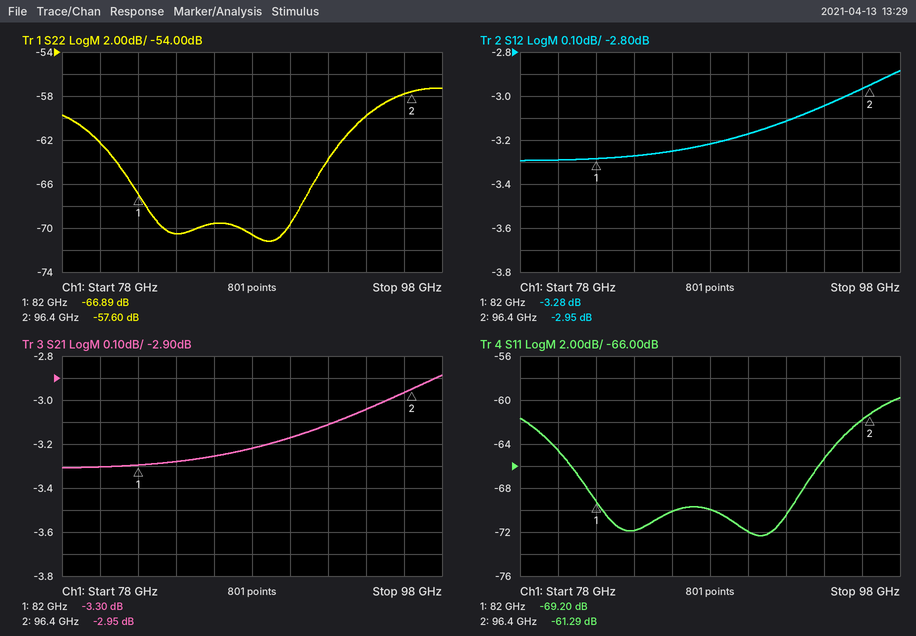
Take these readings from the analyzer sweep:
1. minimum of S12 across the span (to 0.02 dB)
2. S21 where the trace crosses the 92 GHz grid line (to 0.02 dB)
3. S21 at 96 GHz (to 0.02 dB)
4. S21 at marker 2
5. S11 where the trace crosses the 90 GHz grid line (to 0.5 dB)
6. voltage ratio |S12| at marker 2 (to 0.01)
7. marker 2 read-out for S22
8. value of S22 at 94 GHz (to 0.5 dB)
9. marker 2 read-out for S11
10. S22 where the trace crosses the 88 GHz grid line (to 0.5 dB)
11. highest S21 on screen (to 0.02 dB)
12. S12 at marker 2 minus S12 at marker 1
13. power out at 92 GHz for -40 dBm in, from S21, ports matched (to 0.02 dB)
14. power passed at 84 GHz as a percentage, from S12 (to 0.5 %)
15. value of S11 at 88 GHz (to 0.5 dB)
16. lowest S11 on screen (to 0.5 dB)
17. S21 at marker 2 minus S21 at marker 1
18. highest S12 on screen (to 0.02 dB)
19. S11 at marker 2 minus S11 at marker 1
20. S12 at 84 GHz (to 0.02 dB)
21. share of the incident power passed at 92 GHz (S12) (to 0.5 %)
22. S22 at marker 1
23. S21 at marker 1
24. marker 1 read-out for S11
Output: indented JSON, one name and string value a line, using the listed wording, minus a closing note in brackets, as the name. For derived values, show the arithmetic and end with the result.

{
  "minimum of S12 across the span": "-3.30 dB",
  "S21 where the trace crosses the 92 GHz grid line": "-3.12 dB",
  "S21 at 96 GHz": "-2.96 dB",
  "S21 at marker 2": "-2.95 dB",
  "S11 where the trace crosses the 90 GHz grid line": "-72.0 dB",
  "voltage ratio |S12| at marker 2": "10^(-2.95/20) ≈ 0.71",
  "marker 2 read-out for S22": "-57.60 dB",
  "value of S22 at 94 GHz": "-60.0 dB",
  "marker 2 read-out for S11": "-61.29 dB",
  "S22 where the trace crosses the 88 GHz grid line": "-70.5 dB",
  "highest S21 on screen": "-2.88 dB",
  "S12 at marker 2 minus S12 at marker 1": "-2.95 − (-3.28) = 0.33 dB",
  "power out at 92 GHz for -40 dBm in, from S21, ports matched": "-40 dBm + (-3.12 dB) = -43.12 dBm",
  "power passed at 84 GHz as a percentage, from S12": "10^(-3.28/10) ≈ 47.0 %",
  "value of S11 at 88 GHz": "-70.0 dB",
  "lowest S11 on screen": "-72.5 dB",
  "S21 at marker 2 minus S21 at marker 1": "-2.95 − (-3.3) = 0.35 dB",
  "highest S12 on screen": "-2.88 dB",
  "S11 at marker 2 minus S11 at marker 1": "-61.29 − (-69.2) = 7.91 dB",
  "S12 at 84 GHz": "-3.28 dB",
  "share of the incident power passed at 92 GHz (S12)": "10^(-3.12/10) ≈ 48.8 %, so 49.0 % to the nearest 0.5 %",
  "S22 at marker 1": "-66.89 dB",
  "S21 at marker 1": "-3.30 dB",
  "marker 1 read-out for S11": "-69.20 dB"
}
